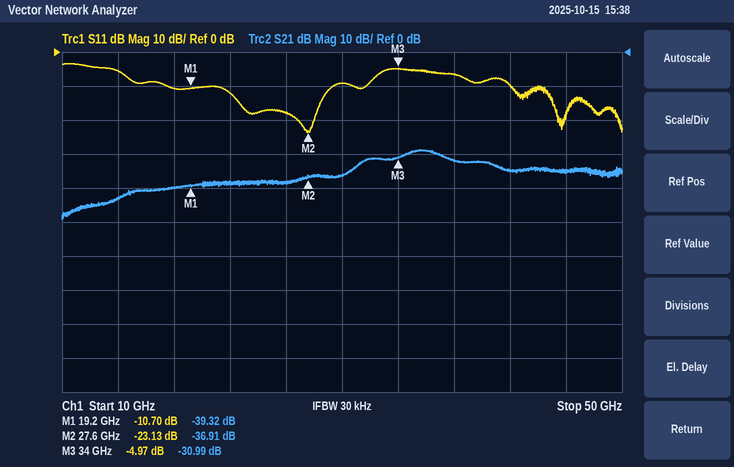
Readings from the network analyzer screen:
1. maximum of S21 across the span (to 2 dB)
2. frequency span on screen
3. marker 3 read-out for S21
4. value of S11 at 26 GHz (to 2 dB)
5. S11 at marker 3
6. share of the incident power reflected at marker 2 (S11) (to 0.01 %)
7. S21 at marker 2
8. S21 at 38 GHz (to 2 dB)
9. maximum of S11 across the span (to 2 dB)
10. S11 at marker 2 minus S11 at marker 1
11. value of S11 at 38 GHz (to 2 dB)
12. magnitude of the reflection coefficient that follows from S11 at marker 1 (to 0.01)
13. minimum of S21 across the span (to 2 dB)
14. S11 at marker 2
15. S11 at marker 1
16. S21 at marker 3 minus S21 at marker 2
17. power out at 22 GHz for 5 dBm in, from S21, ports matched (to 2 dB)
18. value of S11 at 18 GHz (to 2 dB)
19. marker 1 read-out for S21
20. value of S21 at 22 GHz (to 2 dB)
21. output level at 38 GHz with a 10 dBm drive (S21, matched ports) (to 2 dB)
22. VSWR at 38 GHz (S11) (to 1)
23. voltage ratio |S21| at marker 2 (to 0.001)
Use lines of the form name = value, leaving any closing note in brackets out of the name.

maximum of S21 across the span = -28 dB
frequency span on screen = 40 GHz
marker 3 read-out for S21 = -30.99 dB
value of S11 at 26 GHz = -18 dB
S11 at marker 3 = -4.97 dB
share of the incident power reflected at marker 2 (S11) = 0.49 %
S21 at marker 2 = -36.91 dB
S21 at 38 GHz = -32 dB
maximum of S11 across the span = -4 dB
S11 at marker 2 minus S11 at marker 1 = -12.43 dB
value of S11 at 38 GHz = -6 dB
magnitude of the reflection coefficient that follows from S11 at marker 1 = 0.29
minimum of S21 across the span = -50 dB
S11 at marker 2 = -23.13 dB
S11 at marker 1 = -10.70 dB
S21 at marker 3 minus S21 at marker 2 = 5.92 dB
power out at 22 GHz for 5 dBm in, from S21, ports matched = -34 dBm
value of S11 at 18 GHz = -10 dB
marker 1 read-out for S21 = -39.32 dB
value of S21 at 22 GHz = -38 dB
output level at 38 GHz with a 10 dBm drive (S21, matched ports) = -22 dBm
VSWR at 38 GHz (S11) = 3
voltage ratio |S21| at marker 2 = 0.014
